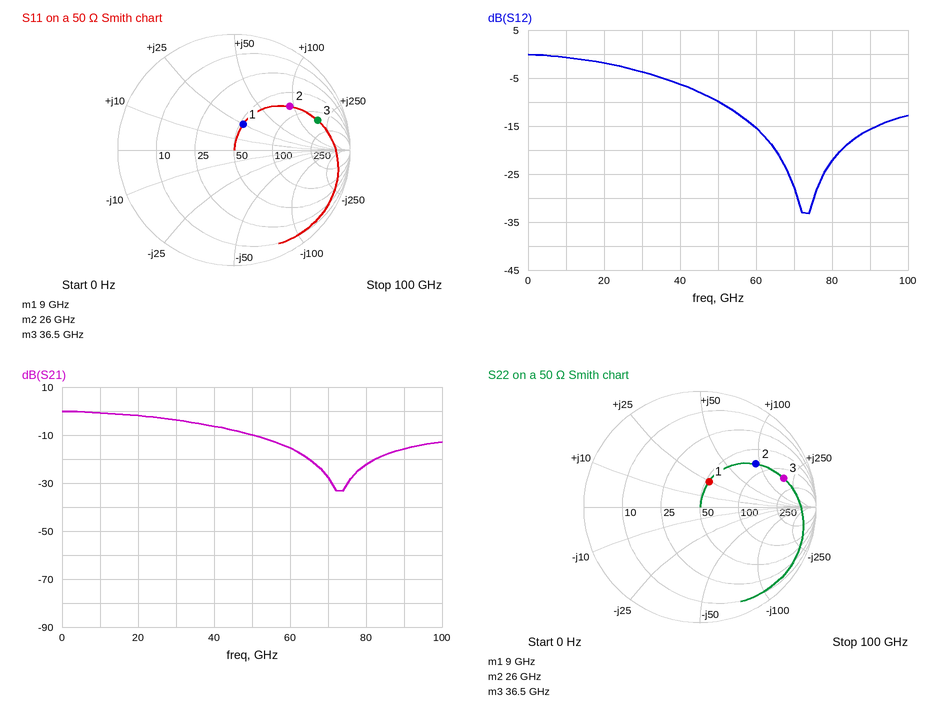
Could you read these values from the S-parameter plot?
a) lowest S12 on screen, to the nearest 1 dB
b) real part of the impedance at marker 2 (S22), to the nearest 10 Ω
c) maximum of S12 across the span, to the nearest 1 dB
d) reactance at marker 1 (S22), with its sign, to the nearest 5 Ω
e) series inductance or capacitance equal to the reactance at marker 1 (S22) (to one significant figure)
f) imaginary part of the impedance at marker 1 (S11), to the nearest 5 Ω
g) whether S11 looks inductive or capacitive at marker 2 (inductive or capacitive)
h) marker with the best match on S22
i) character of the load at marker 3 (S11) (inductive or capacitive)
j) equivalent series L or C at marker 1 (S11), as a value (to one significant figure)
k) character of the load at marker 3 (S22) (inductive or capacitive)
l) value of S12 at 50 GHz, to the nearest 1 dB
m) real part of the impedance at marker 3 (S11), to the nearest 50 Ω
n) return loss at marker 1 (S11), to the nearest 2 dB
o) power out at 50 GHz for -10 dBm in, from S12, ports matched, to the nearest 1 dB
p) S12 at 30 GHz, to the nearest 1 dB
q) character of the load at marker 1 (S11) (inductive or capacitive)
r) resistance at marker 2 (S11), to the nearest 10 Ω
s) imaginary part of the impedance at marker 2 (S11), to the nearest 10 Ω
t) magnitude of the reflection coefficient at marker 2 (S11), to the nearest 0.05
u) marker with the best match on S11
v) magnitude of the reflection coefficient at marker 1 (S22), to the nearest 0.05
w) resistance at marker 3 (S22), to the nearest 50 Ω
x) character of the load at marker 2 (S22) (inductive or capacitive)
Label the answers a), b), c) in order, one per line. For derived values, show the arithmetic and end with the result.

a) -33 dB
b) 80 Ω
c) 0 dB
d) +25 Ω
e) L = 25 Ω/(2π × 9 GHz) ≈ 442 pH, so 400 pH to one significant figure
f) +25 Ω
g) inductive
h) marker 1
i) inductive
j) L = 25 Ω/(2π × 9 GHz) ≈ 442 pH, so 400 pH to one significant figure
k) inductive
l) -10 dB
m) 150 Ω
n) 12 dB
o) -10 dBm + (-10 dB) = -20 dBm
p) -4 dB
q) inductive
r) 80 Ω
s) +90 Ω
t) 0.60
u) marker 1
v) 0.25
w) 150 Ω
x) inductive
